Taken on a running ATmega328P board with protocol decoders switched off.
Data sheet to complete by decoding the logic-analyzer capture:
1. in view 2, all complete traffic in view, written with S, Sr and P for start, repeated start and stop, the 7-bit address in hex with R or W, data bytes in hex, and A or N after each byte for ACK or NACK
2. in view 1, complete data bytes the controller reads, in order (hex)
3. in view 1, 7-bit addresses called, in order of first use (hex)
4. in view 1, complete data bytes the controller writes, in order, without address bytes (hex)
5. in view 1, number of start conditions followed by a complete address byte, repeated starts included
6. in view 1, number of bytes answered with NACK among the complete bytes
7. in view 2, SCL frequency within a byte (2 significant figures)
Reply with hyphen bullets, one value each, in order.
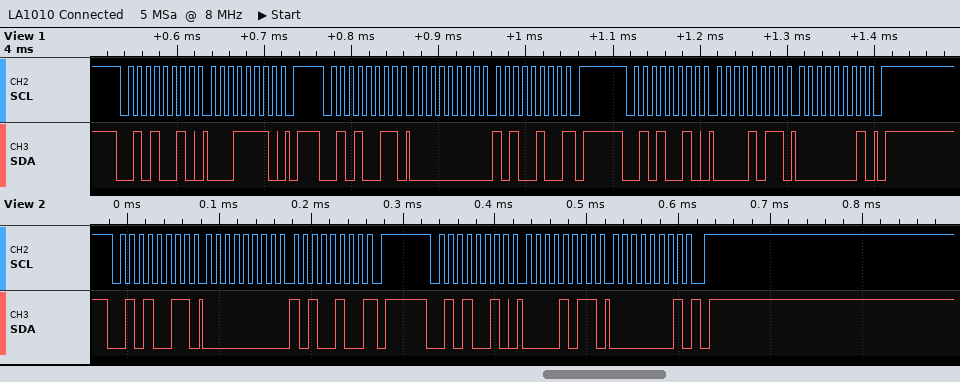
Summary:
- S 29R A 00 A A4 N P S 29W A 0B A 01 A P
- 00 A4
- 0x29
- 1E 0B 01
- 3
- 1
- 100 kHz
